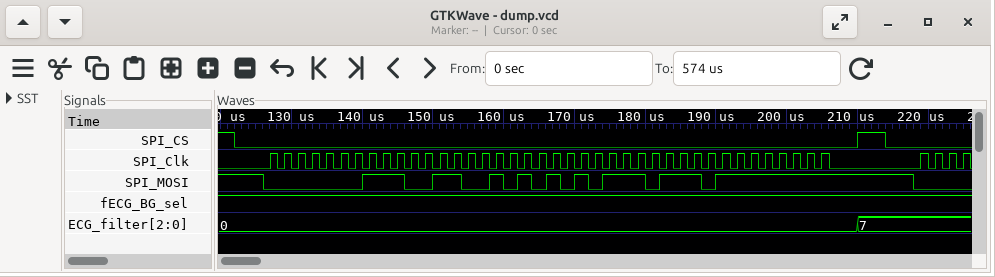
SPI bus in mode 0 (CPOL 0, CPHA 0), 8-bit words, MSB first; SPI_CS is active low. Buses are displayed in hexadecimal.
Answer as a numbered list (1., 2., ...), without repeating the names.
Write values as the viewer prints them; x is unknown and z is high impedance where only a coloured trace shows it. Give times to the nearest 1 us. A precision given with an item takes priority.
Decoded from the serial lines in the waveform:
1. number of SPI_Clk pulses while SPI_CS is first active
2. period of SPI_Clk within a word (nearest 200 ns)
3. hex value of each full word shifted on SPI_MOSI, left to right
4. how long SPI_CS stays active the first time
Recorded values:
1. 40
2. 2000 ns
3. 01, CC, AA, EE, FF
4. 88 us
